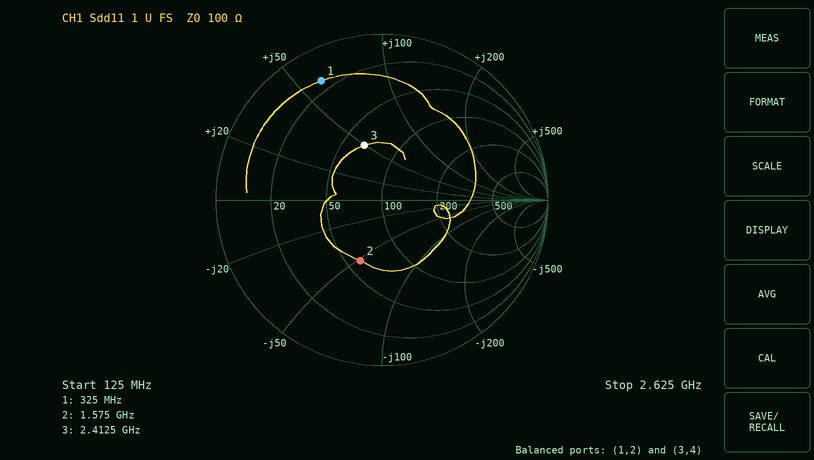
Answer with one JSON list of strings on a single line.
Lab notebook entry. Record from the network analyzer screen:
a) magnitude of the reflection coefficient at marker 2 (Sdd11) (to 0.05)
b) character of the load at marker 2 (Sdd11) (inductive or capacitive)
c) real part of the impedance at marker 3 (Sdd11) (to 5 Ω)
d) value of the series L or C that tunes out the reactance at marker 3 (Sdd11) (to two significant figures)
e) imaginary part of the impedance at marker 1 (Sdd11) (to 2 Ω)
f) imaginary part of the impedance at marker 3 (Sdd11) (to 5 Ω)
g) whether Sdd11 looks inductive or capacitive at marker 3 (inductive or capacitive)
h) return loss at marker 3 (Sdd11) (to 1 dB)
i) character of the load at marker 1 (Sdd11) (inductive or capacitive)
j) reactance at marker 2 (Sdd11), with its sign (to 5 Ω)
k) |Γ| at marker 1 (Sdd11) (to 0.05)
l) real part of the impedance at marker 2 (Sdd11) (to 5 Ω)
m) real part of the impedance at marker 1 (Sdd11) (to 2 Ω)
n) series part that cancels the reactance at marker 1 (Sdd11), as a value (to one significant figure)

["0.40", "capacitive", "65 Ω", "1.3 pF", "+60 Ω", "+50 Ω", "inductive", "9 dB", "inductive", "-50 Ω", "0.80", "60 Ω", "14 Ω", "8 pF"]
